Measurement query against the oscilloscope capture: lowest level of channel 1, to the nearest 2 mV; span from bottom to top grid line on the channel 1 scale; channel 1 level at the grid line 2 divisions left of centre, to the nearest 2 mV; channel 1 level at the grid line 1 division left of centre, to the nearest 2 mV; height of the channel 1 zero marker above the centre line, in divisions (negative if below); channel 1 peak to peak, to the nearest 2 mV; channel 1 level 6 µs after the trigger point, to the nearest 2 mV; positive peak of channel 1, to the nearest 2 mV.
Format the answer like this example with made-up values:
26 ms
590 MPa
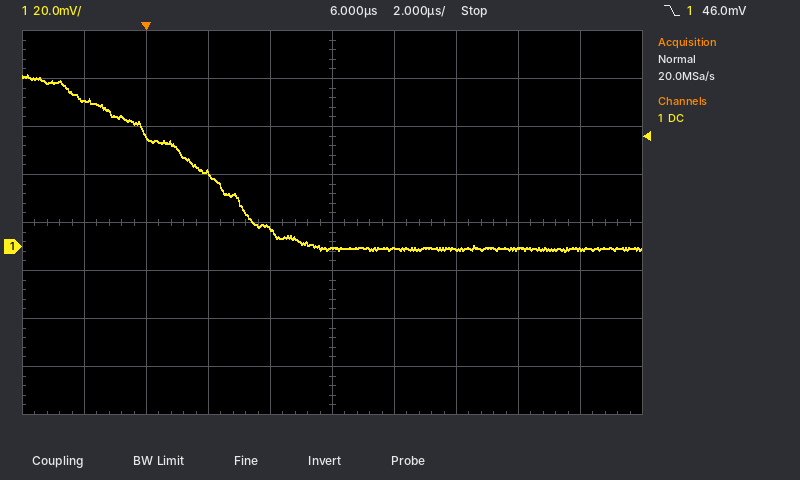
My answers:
-2 mV
160 mV
30 mV
8 mV
-0.5 div
74 mV
0 mV
72 mV
